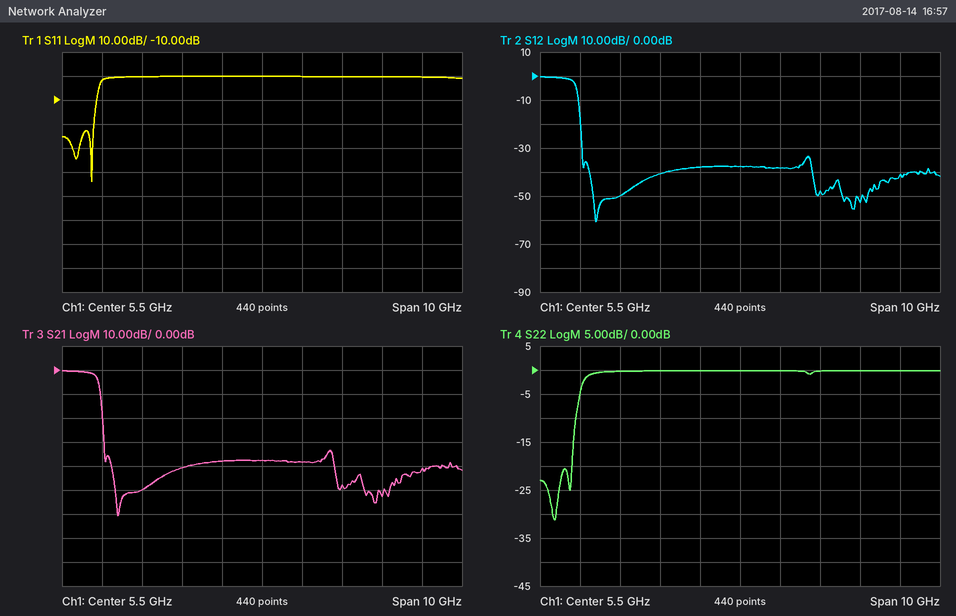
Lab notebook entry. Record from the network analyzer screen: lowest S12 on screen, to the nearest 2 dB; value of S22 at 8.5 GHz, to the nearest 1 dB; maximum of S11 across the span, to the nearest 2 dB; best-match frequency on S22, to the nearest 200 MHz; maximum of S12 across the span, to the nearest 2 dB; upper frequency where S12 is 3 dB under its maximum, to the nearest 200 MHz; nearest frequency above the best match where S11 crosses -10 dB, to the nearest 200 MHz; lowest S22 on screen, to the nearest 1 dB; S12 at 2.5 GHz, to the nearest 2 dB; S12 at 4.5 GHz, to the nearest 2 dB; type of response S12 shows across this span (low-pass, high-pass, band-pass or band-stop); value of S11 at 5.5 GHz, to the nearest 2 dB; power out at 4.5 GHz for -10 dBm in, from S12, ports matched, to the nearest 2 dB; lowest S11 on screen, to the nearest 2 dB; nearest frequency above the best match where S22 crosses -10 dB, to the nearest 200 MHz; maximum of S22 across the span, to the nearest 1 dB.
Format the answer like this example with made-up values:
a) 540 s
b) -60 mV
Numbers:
a) -60 dB
b) 0 dB
c) 0 dB
d) 800 MHz
e) 0 dB
f) 1.4 GHz
g) 1.4 GHz
h) -31 dB
i) -50 dB
j) -38 dB
k) low-pass
l) 0 dB
m) -48 dBm
n) -44 dB
o) 1.4 GHz
p) 0 dB
